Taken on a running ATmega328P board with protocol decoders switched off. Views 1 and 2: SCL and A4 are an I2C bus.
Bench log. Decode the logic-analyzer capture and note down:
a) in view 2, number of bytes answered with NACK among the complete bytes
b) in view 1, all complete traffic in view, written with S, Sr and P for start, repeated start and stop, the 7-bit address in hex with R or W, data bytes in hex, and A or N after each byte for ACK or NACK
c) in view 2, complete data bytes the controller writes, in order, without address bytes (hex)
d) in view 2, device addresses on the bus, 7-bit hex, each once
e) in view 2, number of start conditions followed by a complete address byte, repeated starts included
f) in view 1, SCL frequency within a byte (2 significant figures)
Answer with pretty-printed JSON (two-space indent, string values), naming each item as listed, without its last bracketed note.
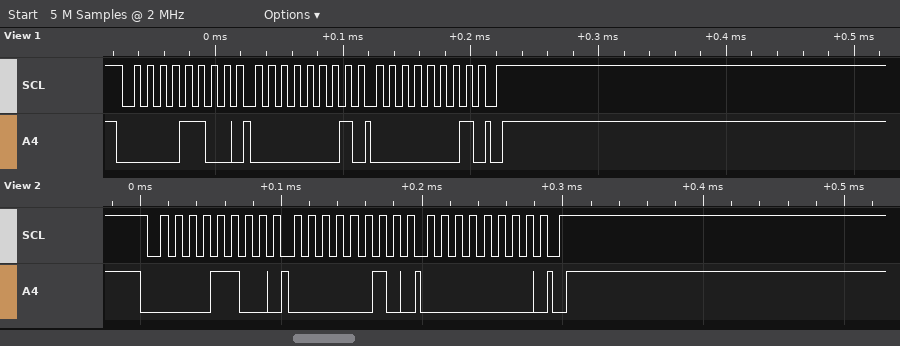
{
  "in view 2, number of bytes answered with NACK among the complete bytes": "0",
  "in view 1, all complete traffic in view, written with S, Sr and P for start, repeated start and stop, the 7-bit address in hex with R or W, data bytes in hex, and A or N after each byte for ACK or NACK": "S 06W A 01 A 01 A P",
  "in view 2, complete data bytes the controller writes, in order, without address bytes": "02 00",
  "in view 2, device addresses on the bus, 7-bit hex, each once": "0x06",
  "in view 2, number of start conditions followed by a complete address byte, repeated starts included": "1",
  "in view 1, SCL frequency within a byte": "100 kHz"
}
